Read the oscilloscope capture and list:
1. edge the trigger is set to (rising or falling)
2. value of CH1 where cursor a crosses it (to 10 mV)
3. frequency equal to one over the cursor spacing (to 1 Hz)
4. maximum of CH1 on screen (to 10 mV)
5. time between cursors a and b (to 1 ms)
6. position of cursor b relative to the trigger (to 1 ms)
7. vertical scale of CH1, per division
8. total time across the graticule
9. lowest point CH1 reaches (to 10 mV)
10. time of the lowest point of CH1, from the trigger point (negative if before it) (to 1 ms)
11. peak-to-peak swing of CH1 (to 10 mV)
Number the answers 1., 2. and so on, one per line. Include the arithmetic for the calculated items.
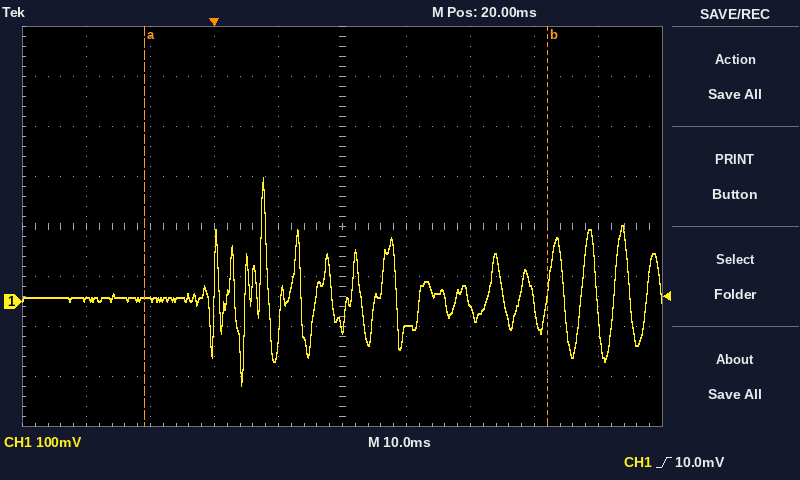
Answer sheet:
1. rising
2. 10 mV
3. 1 / 63 ms ≈ 16 Hz
4. 250 mV
5. 63 ms
6. +52 ms
7. 100 mV
8. 100 ms
9. -170 mV
10. +4 ms
11. 250 mV − (-170 mV) = 420 mV
